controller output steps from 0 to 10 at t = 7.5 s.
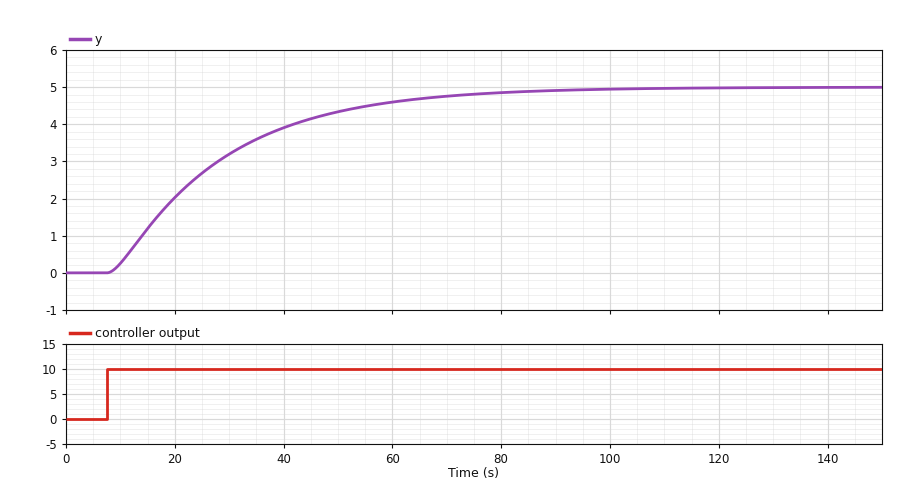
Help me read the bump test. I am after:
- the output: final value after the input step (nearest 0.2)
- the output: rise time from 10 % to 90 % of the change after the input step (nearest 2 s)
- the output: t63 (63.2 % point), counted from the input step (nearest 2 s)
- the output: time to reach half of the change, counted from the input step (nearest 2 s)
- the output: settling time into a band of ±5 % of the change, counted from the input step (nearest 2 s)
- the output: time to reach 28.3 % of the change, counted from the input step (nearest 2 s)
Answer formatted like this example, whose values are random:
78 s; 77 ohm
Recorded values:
5.0; 44 s; 22 s; 16 s; 62 s; 8 s
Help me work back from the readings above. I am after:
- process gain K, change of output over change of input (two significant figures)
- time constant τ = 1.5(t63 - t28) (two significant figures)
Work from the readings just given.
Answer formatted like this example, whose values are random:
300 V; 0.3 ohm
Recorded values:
0.50; 21 s
